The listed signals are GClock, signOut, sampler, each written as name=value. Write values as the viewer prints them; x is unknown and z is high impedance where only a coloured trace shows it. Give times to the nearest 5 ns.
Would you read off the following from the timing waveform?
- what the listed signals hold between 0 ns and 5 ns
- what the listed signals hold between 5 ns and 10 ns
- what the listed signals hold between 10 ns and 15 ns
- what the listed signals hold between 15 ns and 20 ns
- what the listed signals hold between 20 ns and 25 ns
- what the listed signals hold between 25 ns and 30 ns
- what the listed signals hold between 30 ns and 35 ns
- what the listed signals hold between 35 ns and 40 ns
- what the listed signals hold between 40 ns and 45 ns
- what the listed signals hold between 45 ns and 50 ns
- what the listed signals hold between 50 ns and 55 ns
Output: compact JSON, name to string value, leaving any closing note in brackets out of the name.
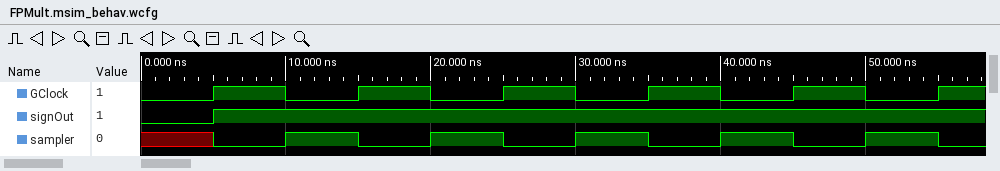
{"what the listed signals hold between 0 ns and 5 ns": "GClock=0, signOut=0, sampler=x", "what the listed signals hold between 5 ns and 10 ns": "GClock=1, signOut=1, sampler=0", "what the listed signals hold between 10 ns and 15 ns": "GClock=0, signOut=1, sampler=1", "what the listed signals hold between 15 ns and 20 ns": "GClock=1, signOut=1, sampler=0", "what the listed signals hold between 20 ns and 25 ns": "GClock=0, signOut=1, sampler=1", "what the listed signals hold between 25 ns and 30 ns": "GClock=1, signOut=1, sampler=0", "what the listed signals hold between 30 ns and 35 ns": "GClock=0, signOut=1, sampler=1", "what the listed signals hold between 35 ns and 40 ns": "GClock=1, signOut=1, sampler=0", "what the listed signals hold between 40 ns and 45 ns": "GClock=0, signOut=1, sampler=1", "what the listed signals hold between 45 ns and 50 ns": "GClock=1, signOut=1, sampler=0", "what the listed signals hold between 50 ns and 55 ns": "GClock=0, signOut=1, sampler=1"}
